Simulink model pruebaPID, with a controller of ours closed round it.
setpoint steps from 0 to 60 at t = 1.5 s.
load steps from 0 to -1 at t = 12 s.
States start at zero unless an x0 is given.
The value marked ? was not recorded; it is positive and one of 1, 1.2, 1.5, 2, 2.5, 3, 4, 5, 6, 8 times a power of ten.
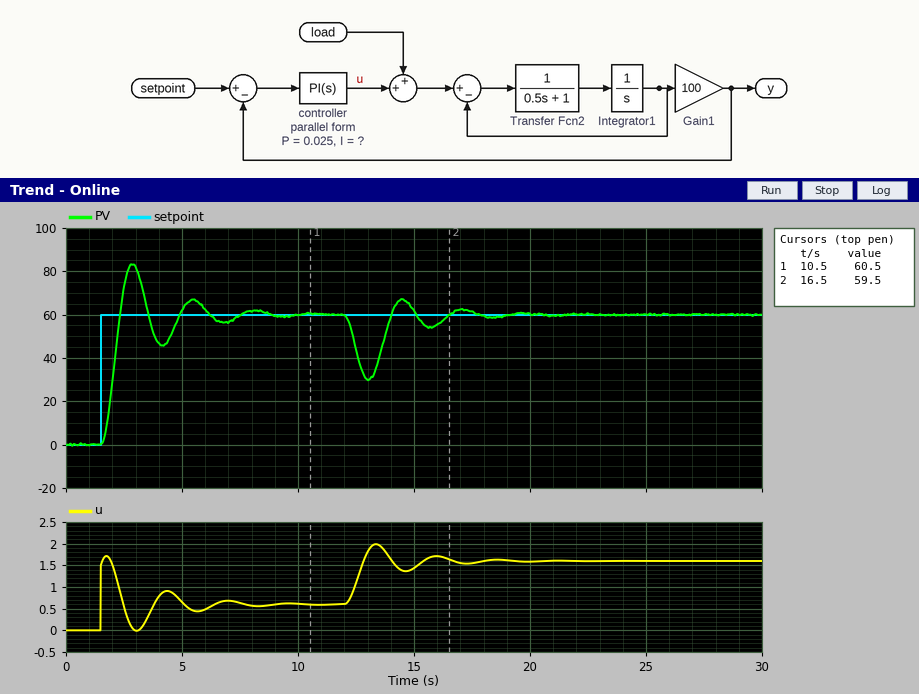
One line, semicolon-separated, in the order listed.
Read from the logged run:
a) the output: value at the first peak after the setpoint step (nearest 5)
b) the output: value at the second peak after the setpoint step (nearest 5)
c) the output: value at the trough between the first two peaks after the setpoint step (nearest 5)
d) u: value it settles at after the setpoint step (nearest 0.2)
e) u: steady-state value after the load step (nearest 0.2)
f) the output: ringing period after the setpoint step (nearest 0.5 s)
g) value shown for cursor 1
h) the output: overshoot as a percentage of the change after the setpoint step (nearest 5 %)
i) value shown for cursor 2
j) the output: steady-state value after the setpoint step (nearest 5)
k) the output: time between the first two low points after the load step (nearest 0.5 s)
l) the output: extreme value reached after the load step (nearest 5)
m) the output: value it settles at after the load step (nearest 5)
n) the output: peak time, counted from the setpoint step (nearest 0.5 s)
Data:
85; 65; 45; 0.6; 1.6; 2.5 s; 60.5; 40 %; 59.5; 60; 2.5 s; 30; 60; 1.5 s
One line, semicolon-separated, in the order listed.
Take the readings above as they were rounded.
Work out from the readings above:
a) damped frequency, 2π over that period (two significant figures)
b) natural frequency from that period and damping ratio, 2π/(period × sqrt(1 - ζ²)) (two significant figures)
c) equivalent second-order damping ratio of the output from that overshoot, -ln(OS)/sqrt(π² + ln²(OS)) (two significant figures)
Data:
2.5 rad/s; 2.6 rad/s; 0.28
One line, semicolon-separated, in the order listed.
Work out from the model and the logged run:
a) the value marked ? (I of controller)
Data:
0.03
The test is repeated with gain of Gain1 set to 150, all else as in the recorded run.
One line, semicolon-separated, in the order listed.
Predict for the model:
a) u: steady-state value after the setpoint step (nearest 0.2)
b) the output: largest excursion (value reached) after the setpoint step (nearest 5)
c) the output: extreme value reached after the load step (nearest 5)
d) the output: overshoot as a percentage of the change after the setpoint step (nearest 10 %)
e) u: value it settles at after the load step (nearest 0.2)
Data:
0.4; 90; 25; 50 %; 1.4
